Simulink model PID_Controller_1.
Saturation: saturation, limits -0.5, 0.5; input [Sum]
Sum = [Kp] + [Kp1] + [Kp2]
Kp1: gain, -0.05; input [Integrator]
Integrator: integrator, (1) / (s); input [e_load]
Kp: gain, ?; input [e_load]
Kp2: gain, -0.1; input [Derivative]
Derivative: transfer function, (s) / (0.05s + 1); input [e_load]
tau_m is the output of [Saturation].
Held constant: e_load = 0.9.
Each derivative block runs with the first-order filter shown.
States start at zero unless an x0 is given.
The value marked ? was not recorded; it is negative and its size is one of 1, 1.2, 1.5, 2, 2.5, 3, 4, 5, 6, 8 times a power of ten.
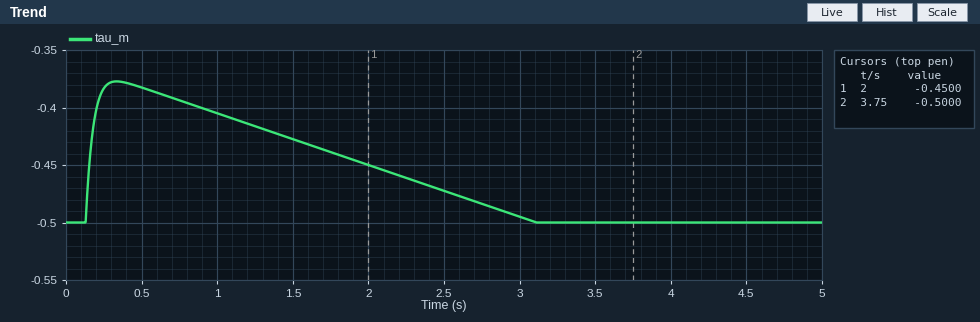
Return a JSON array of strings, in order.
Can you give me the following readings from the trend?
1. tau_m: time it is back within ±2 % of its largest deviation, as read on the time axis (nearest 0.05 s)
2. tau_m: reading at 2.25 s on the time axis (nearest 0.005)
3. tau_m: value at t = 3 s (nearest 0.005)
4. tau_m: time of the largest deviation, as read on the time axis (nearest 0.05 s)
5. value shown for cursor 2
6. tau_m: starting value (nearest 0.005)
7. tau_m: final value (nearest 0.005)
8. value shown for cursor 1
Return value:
["3.05 s", "-0.460", "-0.495", "0.35 s", "-0.5000", "-0.500", "-0.500", "-0.4500"]
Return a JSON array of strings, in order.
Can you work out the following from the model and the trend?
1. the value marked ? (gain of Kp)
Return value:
["-0.4"]
